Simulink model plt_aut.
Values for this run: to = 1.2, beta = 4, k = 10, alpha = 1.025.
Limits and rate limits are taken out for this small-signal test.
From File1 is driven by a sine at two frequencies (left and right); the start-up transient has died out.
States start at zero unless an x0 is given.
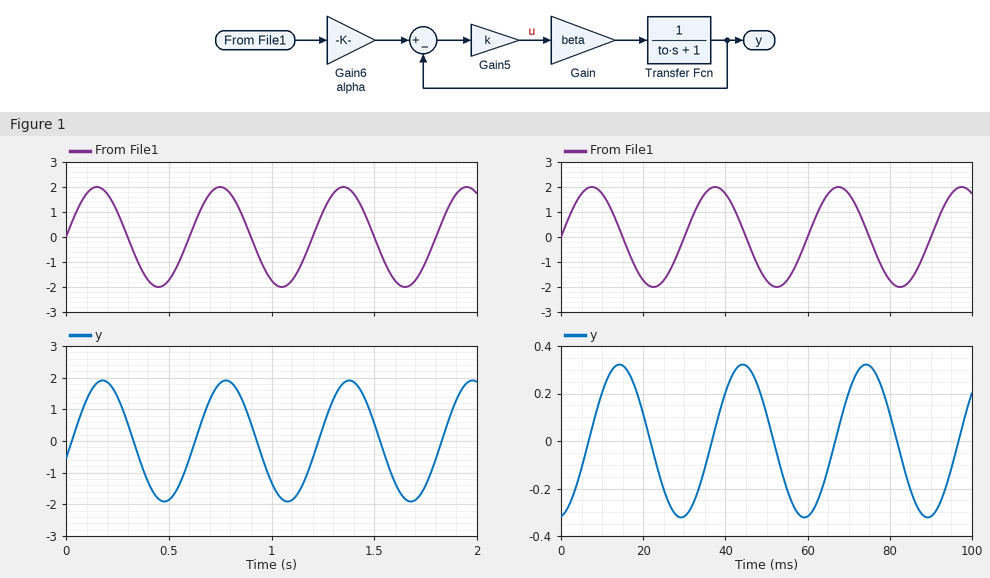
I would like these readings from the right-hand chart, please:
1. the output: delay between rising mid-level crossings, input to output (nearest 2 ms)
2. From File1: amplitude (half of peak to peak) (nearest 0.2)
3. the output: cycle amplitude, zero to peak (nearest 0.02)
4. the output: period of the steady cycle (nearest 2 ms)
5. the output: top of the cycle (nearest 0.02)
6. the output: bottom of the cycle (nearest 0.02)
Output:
6 ms
2.0
0.32
30 ms
0.32
-0.32
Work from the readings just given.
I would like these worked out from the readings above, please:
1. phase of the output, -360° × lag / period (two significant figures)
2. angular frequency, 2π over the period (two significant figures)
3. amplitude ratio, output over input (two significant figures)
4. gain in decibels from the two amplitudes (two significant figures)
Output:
-72°
0.21 rad/ms
0.16
-16 dB
